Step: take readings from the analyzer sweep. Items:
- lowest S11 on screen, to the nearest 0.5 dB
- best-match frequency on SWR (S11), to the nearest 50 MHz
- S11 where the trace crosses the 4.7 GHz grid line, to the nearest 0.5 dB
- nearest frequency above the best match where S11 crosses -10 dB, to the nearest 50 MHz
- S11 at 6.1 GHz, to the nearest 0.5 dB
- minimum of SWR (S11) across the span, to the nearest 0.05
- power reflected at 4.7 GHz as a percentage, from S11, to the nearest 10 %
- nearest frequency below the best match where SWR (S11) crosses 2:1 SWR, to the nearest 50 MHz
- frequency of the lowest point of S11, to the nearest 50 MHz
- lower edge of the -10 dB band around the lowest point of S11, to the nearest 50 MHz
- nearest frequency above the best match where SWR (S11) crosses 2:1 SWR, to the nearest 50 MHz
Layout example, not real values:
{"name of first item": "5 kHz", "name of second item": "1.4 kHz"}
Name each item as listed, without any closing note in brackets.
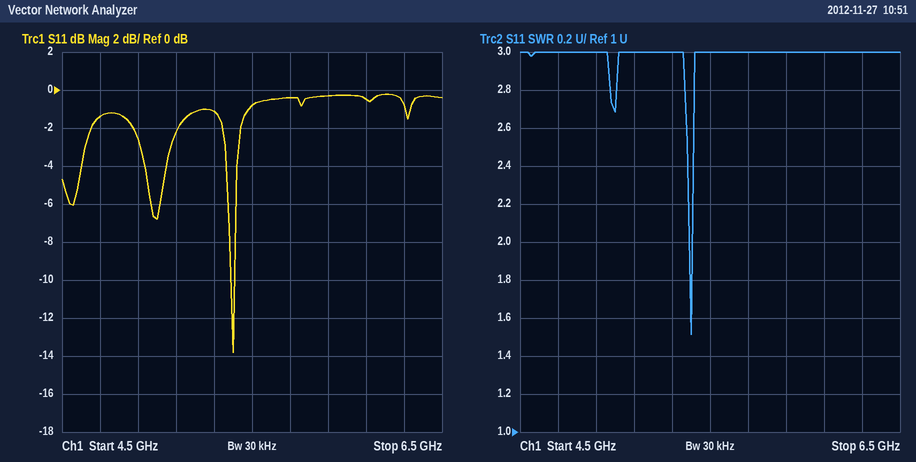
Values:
{"lowest S11 on screen, to the nearest 0.5 dB": "-14.0 dB", "best-match frequency on SWR (S11), to the nearest 50 MHz": "5.40 GHz", "S11 where the trace crosses the 4.7 GHz grid line, to the nearest 0.5 dB": "-1.5 dB", "nearest frequency above the best match where S11 crosses -10 dB, to the nearest 50 MHz": "5.40 GHz", "S11 at 6.1 GHz, to the nearest 0.5 dB": "-0.5 dB", "minimum of SWR (S11) across the span, to the nearest 0.05": "1.50", "power reflected at 4.7 GHz as a percentage, from S11, to the nearest 10 %": "70 %", "nearest frequency below the best match where SWR (S11) crosses 2:1 SWR, to the nearest 50 MHz": "5.40 GHz", "frequency of the lowest point of S11, to the nearest 50 MHz": "5.40 GHz", "lower edge of the -10 dB band around the lowest point of S11, to the nearest 50 MHz": "5.40 GHz", "nearest frequency above the best match where SWR (S11) crosses 2:1 SWR, to the nearest 50 MHz": "5.40 GHz"}
